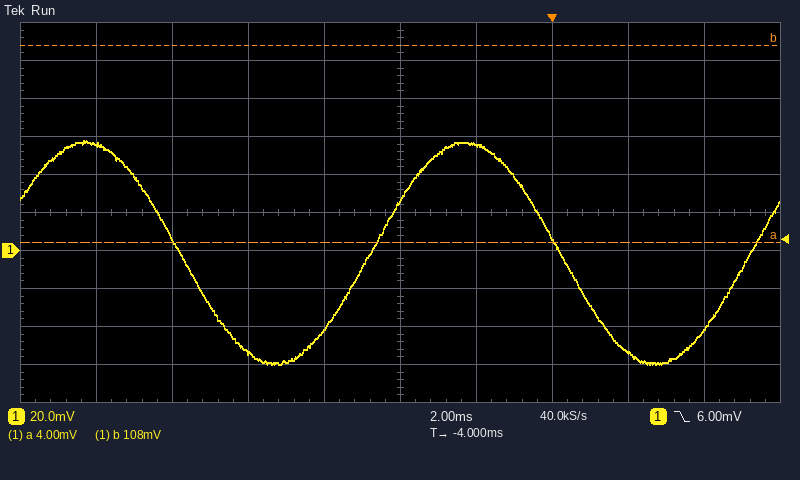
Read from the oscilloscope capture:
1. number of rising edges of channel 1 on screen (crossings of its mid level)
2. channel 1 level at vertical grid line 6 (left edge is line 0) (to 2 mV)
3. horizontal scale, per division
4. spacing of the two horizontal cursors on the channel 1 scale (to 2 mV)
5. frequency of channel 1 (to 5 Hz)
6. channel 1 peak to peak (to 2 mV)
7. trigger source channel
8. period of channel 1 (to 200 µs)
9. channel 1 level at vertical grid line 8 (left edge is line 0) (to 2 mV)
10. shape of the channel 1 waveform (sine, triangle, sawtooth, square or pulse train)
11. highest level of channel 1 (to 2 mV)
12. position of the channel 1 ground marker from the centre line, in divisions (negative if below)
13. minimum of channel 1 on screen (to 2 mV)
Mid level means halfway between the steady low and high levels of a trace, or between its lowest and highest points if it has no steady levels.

2
56 mV
2 ms
104 mV
100 Hz
118 mV
channel 1
10.0 ms
-54 mV
sine
58 mV
-1.0 div
-60 mV
